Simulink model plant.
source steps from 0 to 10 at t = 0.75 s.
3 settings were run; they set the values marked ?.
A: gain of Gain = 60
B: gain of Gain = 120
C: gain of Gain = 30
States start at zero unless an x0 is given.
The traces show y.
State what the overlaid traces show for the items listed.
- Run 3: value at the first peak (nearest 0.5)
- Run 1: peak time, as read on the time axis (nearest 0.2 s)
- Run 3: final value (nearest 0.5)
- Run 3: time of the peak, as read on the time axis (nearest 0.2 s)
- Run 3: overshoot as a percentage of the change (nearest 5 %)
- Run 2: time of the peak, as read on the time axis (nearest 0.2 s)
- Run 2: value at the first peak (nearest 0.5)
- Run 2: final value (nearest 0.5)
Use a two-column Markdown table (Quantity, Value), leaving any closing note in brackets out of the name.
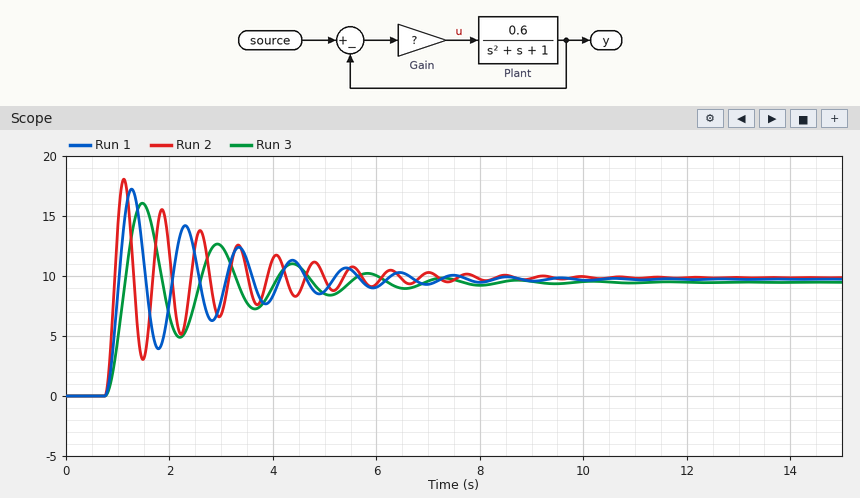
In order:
| Quantity | Value |
|---|---|
| Run 3: value at the first peak | 16.0 |
| Run 1: peak time, as read on the time axis | 1.2 s |
| Run 3: final value | 9.5 |
| Run 3: time of the peak, as read on the time axis | 1.4 s |
| Run 3: overshoot as a percentage of the change | 70 % |
| Run 2: time of the peak, as read on the time axis | 1.2 s |
| Run 2: value at the first peak | 18.0 |
| Run 2: final value | 10.0 |
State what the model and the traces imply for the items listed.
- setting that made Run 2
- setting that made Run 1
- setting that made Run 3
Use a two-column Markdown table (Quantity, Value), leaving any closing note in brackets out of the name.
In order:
| Quantity | Value |
|---|---|
| setting that made Run 2 | B |
| setting that made Run 1 | A |
| setting that made Run 3 | C |
